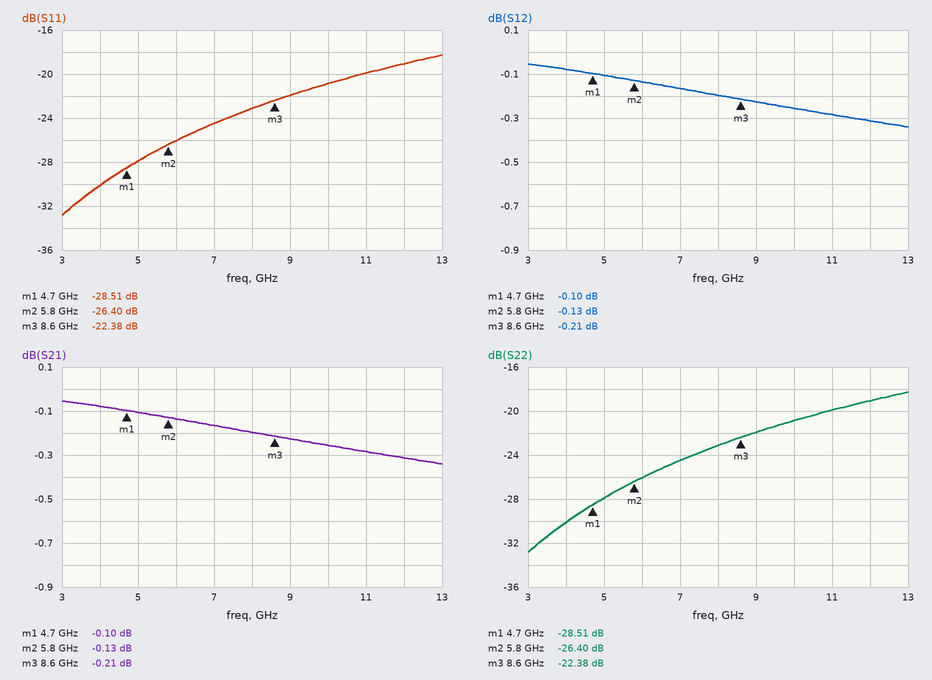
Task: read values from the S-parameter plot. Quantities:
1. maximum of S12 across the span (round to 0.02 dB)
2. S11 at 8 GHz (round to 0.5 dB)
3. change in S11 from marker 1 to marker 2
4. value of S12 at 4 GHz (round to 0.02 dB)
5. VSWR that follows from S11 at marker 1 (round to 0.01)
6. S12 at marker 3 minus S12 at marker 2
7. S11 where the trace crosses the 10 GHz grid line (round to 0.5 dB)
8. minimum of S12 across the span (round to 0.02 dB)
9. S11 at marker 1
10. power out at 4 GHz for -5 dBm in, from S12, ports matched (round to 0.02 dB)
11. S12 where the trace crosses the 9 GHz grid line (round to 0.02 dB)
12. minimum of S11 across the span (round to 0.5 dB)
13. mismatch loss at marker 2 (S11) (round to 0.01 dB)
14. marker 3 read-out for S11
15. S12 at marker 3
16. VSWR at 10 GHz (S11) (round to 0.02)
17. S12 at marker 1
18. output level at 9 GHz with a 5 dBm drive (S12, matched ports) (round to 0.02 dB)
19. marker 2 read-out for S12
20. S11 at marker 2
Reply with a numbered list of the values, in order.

1. -0.06 dB
2. -23.0 dB
3. 2.11 dB
4. -0.08 dB
5. 1.08
6. -0.08 dB
7. -21.0 dB
8. -0.34 dB
9. -28.51 dB
10. -5.08 dBm
11. -0.22 dB
12. -33.0 dB
13. 0.01 dB
14. -22.38 dB
15. -0.21 dB
16. 1.20
17. -0.10 dB
18. 4.78 dBm
19. -0.13 dB
20. -26.40 dB
